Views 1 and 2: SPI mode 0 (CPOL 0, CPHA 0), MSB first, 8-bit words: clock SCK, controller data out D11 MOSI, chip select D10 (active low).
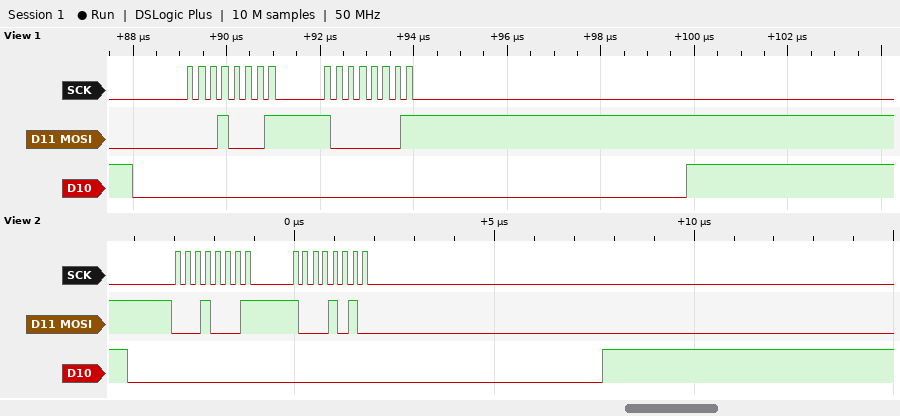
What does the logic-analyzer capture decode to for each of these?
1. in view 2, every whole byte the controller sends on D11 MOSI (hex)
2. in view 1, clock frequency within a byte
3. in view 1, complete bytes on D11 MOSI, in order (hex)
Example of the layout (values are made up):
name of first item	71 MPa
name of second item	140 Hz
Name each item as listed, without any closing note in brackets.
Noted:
in view 2, every whole byte the controller sends on D11 MOSI	11 8A
in view 1, clock frequency within a byte	4 MHz
in view 1, complete bytes on D11 MOSI, in order	11 81
